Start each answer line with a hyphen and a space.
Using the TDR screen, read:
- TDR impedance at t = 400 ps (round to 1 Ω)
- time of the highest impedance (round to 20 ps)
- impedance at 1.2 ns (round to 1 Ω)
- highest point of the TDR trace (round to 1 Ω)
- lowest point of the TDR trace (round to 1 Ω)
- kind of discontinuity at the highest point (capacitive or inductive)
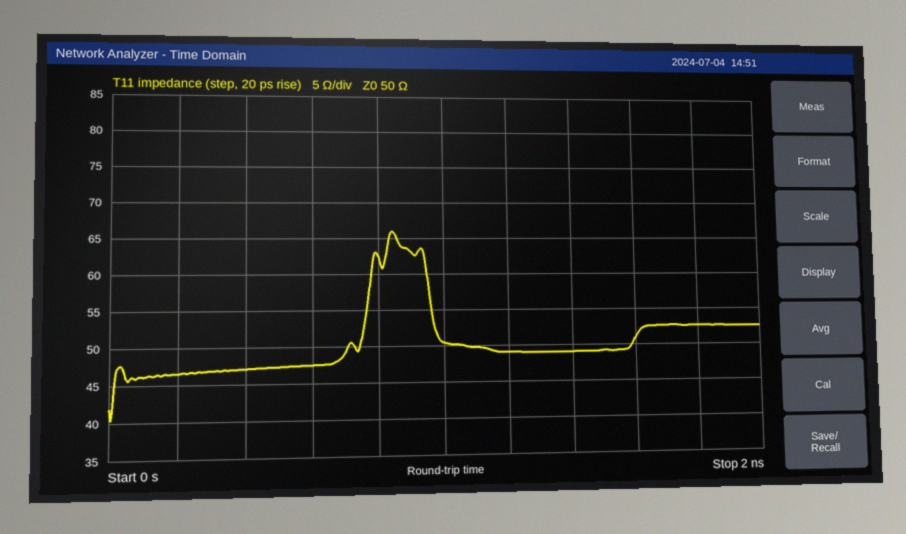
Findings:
- 47 Ω
- 840 ps
- 49 Ω
- 66 Ω
- 40 Ω
- inductive
